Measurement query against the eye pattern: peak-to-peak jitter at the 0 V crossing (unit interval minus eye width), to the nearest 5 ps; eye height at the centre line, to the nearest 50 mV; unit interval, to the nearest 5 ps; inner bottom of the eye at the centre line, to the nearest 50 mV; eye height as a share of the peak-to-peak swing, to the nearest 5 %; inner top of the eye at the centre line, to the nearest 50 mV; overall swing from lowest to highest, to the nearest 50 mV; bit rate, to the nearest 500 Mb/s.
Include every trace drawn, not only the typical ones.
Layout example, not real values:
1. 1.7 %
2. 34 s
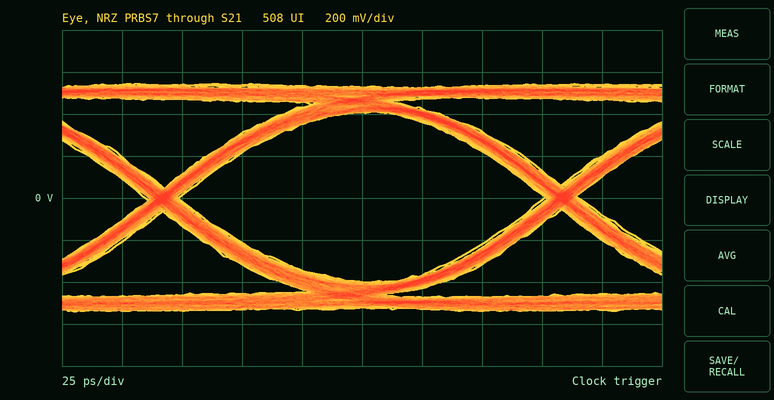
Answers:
1. 15 ps
2. 800 mV
3. 165 ps
4. -400 mV
5. 75 %
6. 400 mV
7. 1.10 V
8. 6.0 Gb/s
